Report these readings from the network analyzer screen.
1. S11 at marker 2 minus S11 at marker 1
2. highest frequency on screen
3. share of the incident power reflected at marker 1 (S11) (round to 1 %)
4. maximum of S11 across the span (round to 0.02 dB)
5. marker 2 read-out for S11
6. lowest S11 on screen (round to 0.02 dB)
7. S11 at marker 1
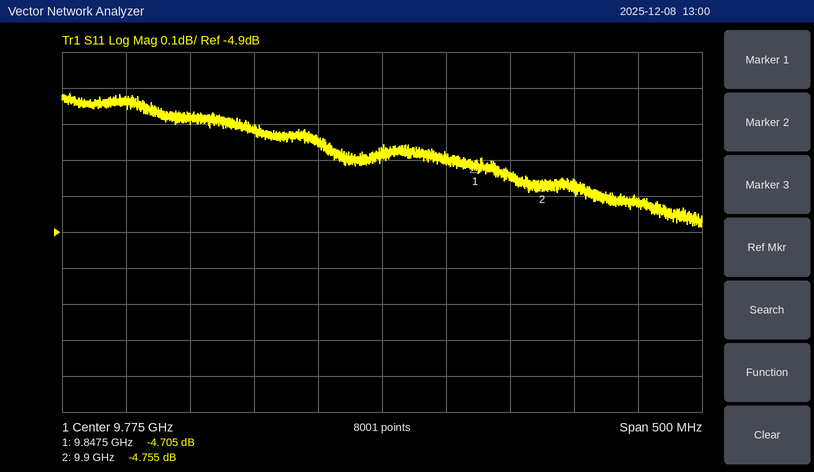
-0.050 dB
10.025 GHz
34 %
-4.52 dB
-4.755 dB
-4.88 dB
-4.705 dB
